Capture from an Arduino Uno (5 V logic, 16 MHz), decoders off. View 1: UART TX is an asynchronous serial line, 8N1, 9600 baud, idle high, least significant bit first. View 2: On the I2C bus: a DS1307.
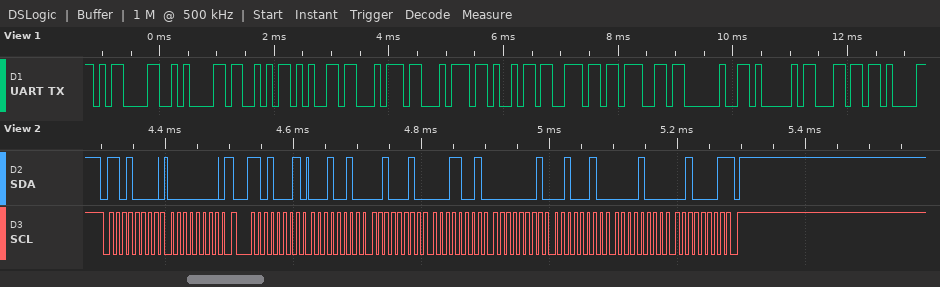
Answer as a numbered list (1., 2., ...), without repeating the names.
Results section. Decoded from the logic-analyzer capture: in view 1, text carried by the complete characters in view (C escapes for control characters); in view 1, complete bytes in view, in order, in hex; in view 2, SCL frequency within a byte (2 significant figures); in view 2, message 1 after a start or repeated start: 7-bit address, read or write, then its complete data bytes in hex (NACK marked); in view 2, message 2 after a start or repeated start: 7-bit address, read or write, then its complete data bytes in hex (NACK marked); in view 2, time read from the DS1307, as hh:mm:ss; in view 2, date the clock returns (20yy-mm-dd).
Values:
1. "\r\nSetting Al"
2. 0x0D 0x0A 0x53 0x65 0x74 0x74 0x69 0x6E 0x67 0x20 0x41 0x6C
3. 100 kHz
4. 0x68 write: 00
5. 0x68 read: 12 22 19 01 22 08 21 NACK
6. 19:22:12
7. 2021-08-22
